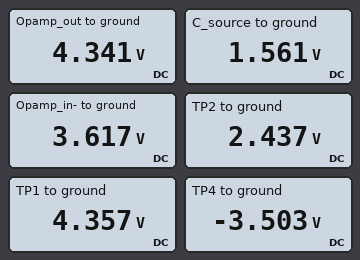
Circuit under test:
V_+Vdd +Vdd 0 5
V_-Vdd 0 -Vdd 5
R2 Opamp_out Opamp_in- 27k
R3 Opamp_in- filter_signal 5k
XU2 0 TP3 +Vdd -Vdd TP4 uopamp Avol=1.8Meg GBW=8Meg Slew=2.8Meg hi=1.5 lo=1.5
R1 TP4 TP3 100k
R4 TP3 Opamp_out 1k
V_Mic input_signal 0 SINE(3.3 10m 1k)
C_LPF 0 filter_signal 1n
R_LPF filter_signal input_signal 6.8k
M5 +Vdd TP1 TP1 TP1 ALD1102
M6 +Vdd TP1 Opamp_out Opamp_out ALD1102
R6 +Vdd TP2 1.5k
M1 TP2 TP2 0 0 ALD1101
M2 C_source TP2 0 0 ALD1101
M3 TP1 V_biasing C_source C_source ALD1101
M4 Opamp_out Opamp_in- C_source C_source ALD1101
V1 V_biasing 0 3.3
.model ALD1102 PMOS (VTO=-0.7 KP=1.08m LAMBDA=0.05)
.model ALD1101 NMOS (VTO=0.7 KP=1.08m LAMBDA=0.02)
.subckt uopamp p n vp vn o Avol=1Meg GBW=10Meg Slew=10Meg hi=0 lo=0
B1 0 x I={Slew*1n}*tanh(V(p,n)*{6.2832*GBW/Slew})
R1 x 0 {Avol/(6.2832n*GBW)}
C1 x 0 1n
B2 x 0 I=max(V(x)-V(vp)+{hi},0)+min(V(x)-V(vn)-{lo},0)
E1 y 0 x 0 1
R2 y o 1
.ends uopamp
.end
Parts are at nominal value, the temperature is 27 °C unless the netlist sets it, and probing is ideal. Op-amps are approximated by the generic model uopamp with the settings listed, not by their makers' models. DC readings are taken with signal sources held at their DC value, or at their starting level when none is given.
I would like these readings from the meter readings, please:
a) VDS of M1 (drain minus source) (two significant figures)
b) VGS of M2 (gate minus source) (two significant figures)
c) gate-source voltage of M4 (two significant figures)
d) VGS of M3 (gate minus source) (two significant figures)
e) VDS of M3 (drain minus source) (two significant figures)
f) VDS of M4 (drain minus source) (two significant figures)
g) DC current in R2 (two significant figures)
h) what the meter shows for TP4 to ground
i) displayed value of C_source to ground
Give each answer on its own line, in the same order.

2.4 V
2.4 V
2.1 V
1.7 V
2.8 V
2.8 V
27 µA
-3.503 V
1.561 V
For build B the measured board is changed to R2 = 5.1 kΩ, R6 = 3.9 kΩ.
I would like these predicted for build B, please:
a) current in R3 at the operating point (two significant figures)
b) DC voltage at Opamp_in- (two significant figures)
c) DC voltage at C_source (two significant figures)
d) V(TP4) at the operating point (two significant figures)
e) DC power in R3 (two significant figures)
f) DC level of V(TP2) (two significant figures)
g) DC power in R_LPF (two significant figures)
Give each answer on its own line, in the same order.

62 µA
4.0 V
2.2 V
-3.5 V
19 µW
1.9 V
26 µW
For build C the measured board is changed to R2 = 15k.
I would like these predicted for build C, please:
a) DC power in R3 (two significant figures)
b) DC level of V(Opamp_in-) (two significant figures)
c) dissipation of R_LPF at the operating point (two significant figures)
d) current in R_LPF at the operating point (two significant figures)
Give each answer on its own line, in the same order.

7.5 µW
3.8 V
10 µW
39 µA
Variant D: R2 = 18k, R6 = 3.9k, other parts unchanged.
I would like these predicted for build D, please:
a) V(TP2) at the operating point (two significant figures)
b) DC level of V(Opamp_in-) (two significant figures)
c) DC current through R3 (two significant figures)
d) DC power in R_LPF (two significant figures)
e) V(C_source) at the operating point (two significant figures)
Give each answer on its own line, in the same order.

1.9 V
3.7 V
35 µA
8.5 µW
2.0 V
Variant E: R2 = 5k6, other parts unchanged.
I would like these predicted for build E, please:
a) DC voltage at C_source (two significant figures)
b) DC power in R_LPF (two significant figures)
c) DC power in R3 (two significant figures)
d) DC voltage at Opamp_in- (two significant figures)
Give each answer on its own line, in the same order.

1.8 V
24 µW
18 µW
4.0 V
